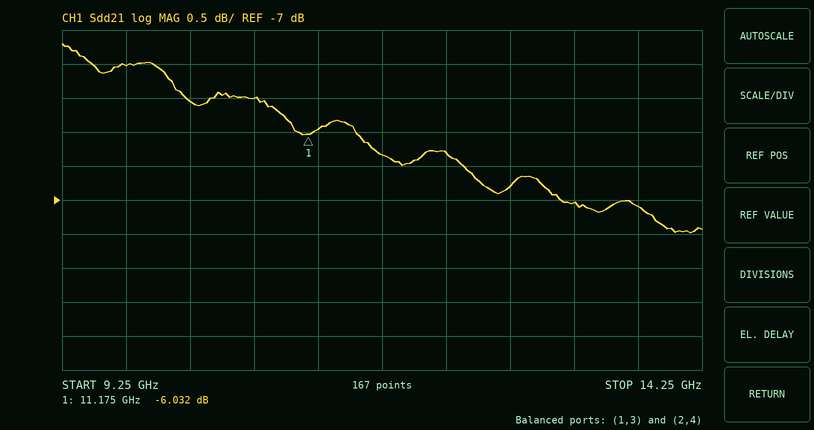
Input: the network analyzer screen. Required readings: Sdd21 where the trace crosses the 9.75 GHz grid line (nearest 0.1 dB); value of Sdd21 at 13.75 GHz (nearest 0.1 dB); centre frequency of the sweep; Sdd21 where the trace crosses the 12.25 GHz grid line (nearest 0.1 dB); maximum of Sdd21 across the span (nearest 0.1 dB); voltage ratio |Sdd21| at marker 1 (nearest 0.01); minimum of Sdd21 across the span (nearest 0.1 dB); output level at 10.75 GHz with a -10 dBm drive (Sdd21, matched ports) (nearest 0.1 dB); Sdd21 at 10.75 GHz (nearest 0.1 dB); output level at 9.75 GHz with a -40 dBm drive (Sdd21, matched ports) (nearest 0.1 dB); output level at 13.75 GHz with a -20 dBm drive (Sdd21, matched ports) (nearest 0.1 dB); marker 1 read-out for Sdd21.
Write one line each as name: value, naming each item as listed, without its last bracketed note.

Sdd21 where the trace crosses the 9.75 GHz grid line: -5.0 dB
value of Sdd21 at 13.75 GHz: -7.1 dB
centre frequency of the sweep: 11.75 GHz
Sdd21 where the trace crosses the 12.25 GHz grid line: -6.3 dB
maximum of Sdd21 across the span: -4.7 dB
voltage ratio |Sdd21| at marker 1: 0.50
minimum of Sdd21 across the span: -7.5 dB
output level at 10.75 GHz with a -10 dBm drive (Sdd21, matched ports): -15.5 dBm
Sdd21 at 10.75 GHz: -5.5 dB
output level at 9.75 GHz with a -40 dBm drive (Sdd21, matched ports): -45.0 dBm
output level at 13.75 GHz with a -20 dBm drive (Sdd21, matched ports): -27.1 dBm
marker 1 read-out for Sdd21: -6.032 dB
